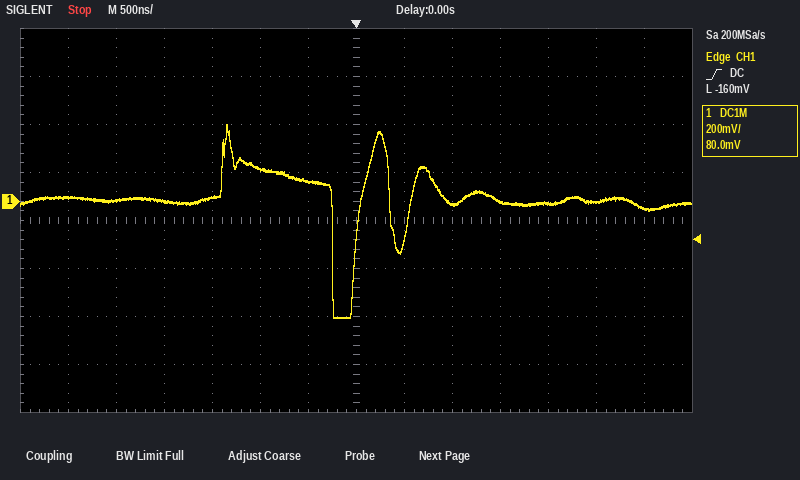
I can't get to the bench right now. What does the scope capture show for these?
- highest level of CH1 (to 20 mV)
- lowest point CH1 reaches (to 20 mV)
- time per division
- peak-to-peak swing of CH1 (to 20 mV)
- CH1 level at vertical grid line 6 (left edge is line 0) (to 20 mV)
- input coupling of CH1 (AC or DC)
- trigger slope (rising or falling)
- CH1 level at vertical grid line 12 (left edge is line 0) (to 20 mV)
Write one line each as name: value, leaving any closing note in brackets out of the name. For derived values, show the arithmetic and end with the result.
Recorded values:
highest level of CH1: 320 mV
lowest point CH1 reaches: -480 mV
time per division: 500 ns
peak-to-peak swing of CH1: 320 mV − (-480 mV) = 800 mV
CH1 level at vertical grid line 6 (left edge is line 0): 80 mV
input coupling of CH1: DC
trigger slope: rising
CH1 level at vertical grid line 12 (left edge is line 0): 0 mV
